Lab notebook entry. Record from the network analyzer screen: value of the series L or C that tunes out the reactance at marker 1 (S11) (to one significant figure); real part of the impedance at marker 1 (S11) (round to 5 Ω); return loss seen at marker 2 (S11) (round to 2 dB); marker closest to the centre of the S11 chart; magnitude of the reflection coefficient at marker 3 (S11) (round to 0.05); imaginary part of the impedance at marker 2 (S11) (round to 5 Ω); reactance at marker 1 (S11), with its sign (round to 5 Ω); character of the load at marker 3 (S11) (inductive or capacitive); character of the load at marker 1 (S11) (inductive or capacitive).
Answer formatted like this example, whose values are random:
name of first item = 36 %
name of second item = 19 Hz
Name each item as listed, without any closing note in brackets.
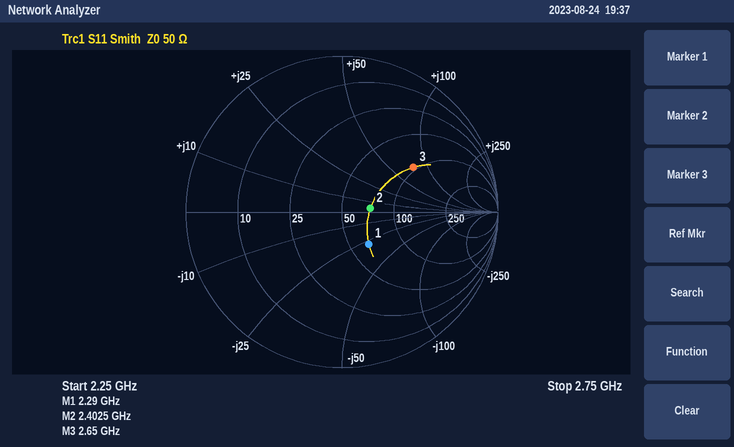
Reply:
value of the series L or C that tunes out the reactance at marker 1 (S11) = 2 nH
real part of the impedance at marker 1 (S11) = 65 Ω
return loss seen at marker 2 (S11) = 14 dB
marker closest to the centre of the S11 chart = marker 2
magnitude of the reflection coefficient at marker 3 (S11) = 0.55
imaginary part of the impedance at marker 2 (S11) = +5 Ω
reactance at marker 1 (S11), with its sign = -30 Ω
character of the load at marker 3 (S11) = inductive
character of the load at marker 1 (S11) = capacitive
